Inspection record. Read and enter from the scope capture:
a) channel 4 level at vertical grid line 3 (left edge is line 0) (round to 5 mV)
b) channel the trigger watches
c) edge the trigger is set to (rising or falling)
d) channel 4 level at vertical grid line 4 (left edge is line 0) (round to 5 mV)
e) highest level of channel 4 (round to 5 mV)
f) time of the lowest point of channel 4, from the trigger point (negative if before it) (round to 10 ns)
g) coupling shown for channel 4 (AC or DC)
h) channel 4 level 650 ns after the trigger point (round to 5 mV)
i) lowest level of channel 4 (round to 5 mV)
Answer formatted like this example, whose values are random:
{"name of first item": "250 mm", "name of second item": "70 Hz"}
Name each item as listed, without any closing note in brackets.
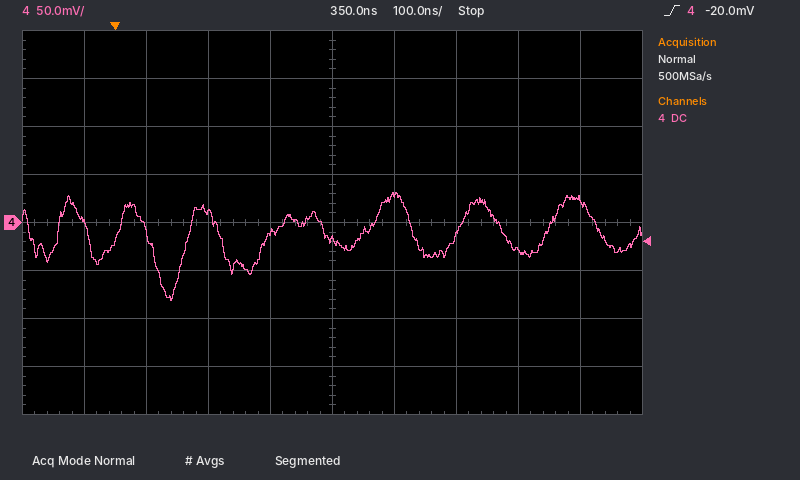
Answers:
{"channel 4 level at vertical grid line 3 (left edge is line 0)": "10 mV", "channel the trigger watches": "channel 4", "edge the trigger is set to": "rising", "channel 4 level at vertical grid line 4 (left edge is line 0)": "-10 mV", "highest level of channel 4": "30 mV", "time of the lowest point of channel 4, from the trigger point (negative if before it)": "+90 ns", "coupling shown for channel 4": "DC", "channel 4 level 650 ns after the trigger point": "-30 mV", "lowest level of channel 4": "-80 mV"}
